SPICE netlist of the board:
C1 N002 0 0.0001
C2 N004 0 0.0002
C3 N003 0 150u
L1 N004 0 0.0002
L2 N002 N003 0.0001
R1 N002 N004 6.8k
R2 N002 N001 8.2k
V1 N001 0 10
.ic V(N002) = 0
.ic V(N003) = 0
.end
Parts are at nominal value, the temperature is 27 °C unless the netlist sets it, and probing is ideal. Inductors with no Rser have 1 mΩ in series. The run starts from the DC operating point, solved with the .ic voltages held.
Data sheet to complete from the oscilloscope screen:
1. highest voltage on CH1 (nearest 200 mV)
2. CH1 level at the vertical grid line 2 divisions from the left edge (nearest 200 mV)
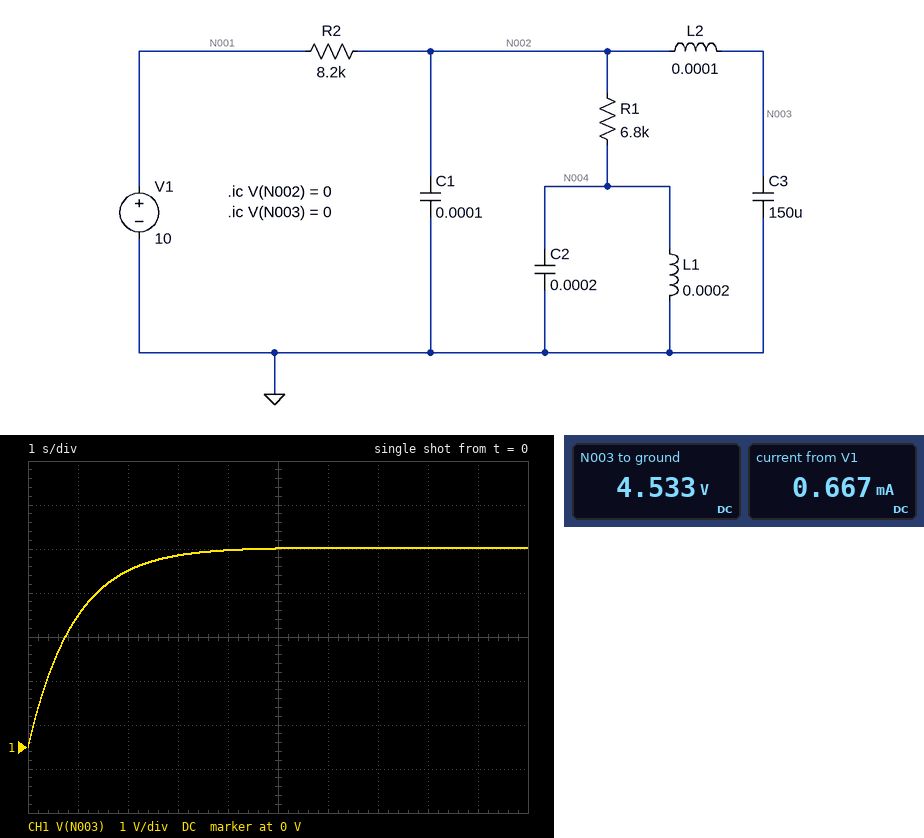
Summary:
4.6 V
4.0 V
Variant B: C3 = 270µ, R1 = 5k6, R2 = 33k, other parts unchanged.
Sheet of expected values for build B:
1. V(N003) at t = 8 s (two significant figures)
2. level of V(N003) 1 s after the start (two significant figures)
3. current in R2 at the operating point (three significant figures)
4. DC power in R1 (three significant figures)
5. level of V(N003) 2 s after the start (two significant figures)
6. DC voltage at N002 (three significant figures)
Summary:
1.4 V
630 mV
259 µA
376 µW
980 mV
1.45 V
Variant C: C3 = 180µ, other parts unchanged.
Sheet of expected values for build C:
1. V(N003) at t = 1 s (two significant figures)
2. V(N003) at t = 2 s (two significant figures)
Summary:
2.8 V
3.9 V
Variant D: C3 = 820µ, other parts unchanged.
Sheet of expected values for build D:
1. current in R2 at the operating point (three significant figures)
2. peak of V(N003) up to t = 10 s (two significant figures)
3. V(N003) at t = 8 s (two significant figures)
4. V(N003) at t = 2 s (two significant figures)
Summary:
667 µA
4.3 V
4.1 V
2.0 V
